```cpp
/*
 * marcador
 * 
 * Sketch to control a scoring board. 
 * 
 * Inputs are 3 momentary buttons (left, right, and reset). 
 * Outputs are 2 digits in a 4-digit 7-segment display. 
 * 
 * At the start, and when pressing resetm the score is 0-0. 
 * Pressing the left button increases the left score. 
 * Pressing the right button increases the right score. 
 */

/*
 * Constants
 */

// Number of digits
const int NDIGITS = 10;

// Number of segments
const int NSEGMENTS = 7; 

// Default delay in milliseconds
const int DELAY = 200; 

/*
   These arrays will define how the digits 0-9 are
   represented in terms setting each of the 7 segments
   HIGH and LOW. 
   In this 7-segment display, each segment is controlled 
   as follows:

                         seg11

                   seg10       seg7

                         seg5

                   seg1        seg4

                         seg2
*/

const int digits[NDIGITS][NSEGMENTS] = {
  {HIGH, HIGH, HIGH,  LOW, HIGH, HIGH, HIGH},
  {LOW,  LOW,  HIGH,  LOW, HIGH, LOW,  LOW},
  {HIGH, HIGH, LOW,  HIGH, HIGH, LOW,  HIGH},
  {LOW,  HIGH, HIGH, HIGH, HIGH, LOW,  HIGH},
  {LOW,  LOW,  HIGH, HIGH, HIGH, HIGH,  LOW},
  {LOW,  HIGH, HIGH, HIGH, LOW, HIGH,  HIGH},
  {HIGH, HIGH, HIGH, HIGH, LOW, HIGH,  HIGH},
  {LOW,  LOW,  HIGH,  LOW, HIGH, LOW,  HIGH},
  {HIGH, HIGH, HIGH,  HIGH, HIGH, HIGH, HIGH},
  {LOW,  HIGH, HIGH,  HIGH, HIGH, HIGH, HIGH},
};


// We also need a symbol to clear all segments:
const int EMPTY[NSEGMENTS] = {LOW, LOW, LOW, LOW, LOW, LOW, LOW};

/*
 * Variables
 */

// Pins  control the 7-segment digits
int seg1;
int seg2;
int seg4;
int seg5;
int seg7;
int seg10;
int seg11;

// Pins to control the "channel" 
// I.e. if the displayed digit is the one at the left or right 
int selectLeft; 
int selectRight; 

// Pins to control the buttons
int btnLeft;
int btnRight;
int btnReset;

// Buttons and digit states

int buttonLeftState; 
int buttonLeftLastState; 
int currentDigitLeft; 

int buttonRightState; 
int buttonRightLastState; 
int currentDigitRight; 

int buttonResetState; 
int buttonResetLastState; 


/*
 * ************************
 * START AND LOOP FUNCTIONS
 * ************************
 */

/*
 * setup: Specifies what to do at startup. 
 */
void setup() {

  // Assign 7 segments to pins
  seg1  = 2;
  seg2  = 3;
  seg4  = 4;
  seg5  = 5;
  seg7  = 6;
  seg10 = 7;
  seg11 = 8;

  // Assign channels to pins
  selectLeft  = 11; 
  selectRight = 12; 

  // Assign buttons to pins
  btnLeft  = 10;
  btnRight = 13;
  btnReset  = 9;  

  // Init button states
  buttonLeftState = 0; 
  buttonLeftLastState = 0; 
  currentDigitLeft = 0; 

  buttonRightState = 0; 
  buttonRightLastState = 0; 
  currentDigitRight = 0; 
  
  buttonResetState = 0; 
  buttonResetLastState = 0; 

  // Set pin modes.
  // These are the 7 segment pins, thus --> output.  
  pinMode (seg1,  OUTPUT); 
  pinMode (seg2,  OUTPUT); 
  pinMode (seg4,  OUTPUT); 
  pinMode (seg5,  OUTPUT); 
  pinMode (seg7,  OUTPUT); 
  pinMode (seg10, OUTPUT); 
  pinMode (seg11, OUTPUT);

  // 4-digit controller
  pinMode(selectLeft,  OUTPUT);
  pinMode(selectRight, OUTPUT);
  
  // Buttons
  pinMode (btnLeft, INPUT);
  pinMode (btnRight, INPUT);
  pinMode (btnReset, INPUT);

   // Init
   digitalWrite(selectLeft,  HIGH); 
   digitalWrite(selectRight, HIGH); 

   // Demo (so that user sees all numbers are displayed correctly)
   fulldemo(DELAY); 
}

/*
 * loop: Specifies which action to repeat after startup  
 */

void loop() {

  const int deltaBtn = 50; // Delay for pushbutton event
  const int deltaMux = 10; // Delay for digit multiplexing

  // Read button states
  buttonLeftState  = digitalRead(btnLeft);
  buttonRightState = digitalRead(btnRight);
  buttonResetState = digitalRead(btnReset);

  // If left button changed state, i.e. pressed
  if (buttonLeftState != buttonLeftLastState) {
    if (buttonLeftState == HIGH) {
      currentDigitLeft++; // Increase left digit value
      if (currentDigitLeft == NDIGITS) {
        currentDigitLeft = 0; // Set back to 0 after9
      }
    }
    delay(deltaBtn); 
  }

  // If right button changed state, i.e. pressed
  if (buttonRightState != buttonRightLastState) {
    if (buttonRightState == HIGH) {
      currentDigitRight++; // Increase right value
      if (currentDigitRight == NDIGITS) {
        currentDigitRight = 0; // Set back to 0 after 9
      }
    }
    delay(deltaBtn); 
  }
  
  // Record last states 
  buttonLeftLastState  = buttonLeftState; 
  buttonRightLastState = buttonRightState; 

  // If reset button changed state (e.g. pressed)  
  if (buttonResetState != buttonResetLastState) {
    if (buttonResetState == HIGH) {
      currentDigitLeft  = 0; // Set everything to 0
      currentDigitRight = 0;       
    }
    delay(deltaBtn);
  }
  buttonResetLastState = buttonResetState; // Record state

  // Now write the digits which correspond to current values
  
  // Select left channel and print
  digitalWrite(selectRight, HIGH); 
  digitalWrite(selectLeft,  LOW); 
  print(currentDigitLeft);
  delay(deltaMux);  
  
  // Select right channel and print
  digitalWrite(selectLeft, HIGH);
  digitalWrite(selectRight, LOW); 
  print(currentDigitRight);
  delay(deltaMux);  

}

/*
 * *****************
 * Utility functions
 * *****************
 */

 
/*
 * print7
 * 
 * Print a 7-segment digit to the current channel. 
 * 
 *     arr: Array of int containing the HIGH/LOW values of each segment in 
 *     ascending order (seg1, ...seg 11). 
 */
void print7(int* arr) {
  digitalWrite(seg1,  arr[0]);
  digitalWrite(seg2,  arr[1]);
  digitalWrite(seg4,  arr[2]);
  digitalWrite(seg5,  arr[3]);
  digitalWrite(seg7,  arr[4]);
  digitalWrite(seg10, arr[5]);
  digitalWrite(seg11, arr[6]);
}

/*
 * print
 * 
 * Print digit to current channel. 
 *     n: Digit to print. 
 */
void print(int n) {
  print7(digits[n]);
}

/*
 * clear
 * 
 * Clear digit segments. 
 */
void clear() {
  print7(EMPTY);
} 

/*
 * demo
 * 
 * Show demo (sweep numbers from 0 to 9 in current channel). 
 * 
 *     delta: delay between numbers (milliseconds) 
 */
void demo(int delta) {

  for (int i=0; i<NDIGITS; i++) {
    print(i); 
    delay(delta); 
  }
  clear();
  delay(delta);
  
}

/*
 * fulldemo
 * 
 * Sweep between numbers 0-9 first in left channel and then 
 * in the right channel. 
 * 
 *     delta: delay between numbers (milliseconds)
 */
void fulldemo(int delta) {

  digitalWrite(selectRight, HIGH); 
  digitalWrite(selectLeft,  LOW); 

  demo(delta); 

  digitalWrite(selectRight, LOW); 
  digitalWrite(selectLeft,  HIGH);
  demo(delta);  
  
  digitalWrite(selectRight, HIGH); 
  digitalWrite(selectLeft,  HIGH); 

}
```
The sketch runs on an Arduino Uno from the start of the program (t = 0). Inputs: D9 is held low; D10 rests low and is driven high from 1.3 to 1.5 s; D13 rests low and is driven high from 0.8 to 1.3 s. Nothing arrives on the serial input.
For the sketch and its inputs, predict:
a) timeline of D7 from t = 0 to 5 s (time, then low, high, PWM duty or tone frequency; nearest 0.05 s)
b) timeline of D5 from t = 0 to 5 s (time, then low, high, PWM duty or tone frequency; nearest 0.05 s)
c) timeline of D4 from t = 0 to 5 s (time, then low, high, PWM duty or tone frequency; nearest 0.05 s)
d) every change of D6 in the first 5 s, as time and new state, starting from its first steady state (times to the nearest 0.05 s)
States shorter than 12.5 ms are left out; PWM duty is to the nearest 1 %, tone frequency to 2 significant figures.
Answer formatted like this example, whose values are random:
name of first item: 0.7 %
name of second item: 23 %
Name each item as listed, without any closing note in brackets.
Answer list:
timeline of D7 from t = 0 to 5 s: 0 s high; 0.2 s low; 0.8 s high; 1.4 s low; 1.6 s high; 2 s low; 2.2 s high; 2.4 s low; 3 s high; 3.6 s low; 3.8 s high; 4.2 s low; 4.4 s high
timeline of D5 from t = 0 to 5 s: 0 s low; 0.4 s high; 1.4 s low; 1.6 s high; 2 s low; 2.6 s high; 3.6 s low; 3.8 s high; 4.2 s low
timeline of D4 from t = 0 to 5 s: 0 s high; 0.4 s low; 0.6 s high; 2 s low; 2.2 s high; 2.6 s low; 2.8 s high; 4.2 s low; 4.4 s high
every change of D6 in the first 5 s, as time and new state, starting from its first steady state: 0 s high; 1 s low; 1.4 s high; 2 s low; 2.2 s high; 3.2 s low; 3.6 s high; 4.2 s low; 4.4 s high
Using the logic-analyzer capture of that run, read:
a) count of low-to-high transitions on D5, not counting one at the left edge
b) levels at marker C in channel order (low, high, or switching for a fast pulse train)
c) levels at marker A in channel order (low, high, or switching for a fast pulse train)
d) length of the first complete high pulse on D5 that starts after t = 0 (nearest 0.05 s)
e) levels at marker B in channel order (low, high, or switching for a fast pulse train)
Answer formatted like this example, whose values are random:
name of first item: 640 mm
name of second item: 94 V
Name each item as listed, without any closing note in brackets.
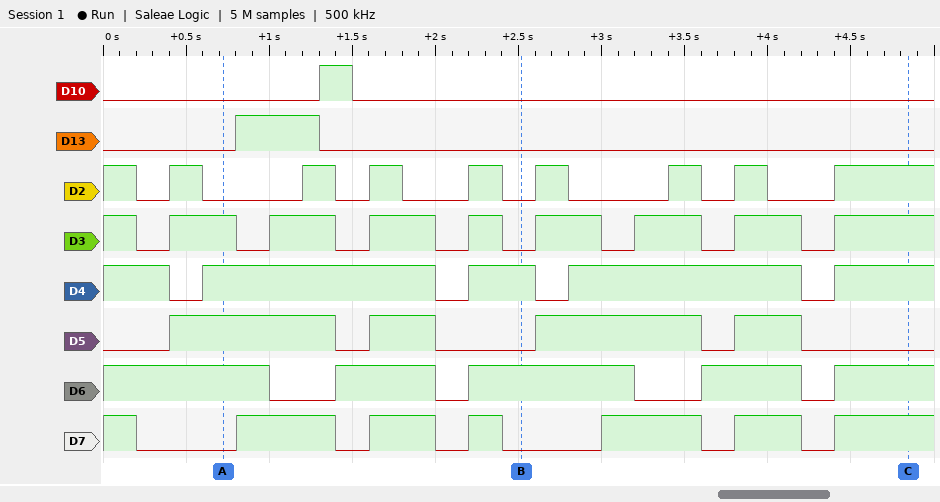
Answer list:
count of low-to-high transitions on D5, not counting one at the left edge: 4
levels at marker C in channel order: D10 low, D13 low, D2 high, D3 high, D4 high, D5 low, D6 high, D7 high
levels at marker A in channel order: D10 low, D13 low, D2 low, D3 high, D4 high, D5 high, D6 high, D7 low
length of the first complete high pulse on D5 that starts after t = 0: 1.00 s
levels at marker B in channel order: D10 low, D13 low, D2 low, D3 low, D4 high, D5 low, D6 high, D7 low
